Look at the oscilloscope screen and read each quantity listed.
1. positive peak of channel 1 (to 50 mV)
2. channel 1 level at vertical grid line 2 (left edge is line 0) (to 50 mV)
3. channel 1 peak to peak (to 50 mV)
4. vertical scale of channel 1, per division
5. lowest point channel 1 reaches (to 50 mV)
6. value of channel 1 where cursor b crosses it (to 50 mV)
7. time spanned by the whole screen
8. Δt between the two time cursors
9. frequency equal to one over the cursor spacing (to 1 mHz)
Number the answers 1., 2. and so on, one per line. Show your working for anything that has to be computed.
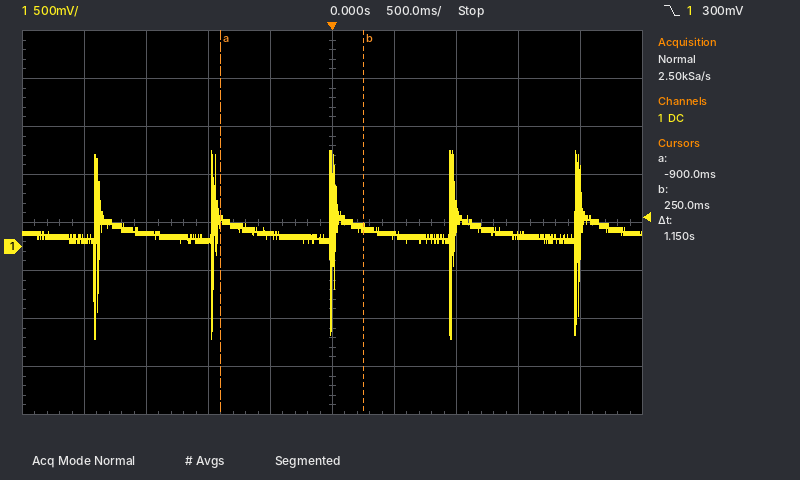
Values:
1. 1.00 V
2. 150 mV
3. 1.00 V − (-950 mV) = 1.95 V
4. 500 mV
5. -950 mV
6. 200 mV
7. 5 s
8. 1.15 s
9. 1 / 1.15 s ≈ 870 mHz
